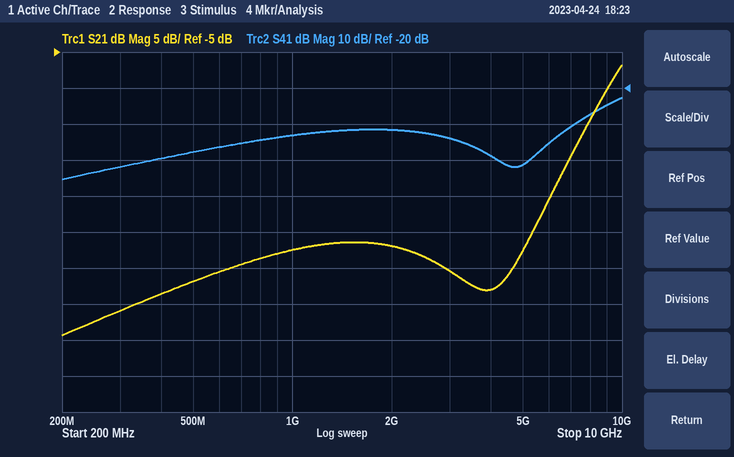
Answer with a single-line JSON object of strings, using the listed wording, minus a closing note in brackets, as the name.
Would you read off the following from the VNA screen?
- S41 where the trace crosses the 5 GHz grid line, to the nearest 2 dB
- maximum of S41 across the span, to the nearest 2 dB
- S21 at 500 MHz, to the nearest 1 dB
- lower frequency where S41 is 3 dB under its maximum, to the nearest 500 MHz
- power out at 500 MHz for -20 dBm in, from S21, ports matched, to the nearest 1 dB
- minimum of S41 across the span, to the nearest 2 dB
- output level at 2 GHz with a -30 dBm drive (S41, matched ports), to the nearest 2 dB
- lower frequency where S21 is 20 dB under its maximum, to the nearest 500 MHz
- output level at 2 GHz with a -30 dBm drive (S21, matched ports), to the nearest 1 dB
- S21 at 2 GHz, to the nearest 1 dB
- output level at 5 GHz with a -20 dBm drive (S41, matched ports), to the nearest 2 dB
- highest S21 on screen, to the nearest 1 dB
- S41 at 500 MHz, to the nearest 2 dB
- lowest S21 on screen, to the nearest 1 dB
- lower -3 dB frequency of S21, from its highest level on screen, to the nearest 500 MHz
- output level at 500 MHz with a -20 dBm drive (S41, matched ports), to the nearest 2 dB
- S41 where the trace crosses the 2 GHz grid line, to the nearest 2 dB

{"S41 where the trace crosses the 5 GHz grid line, to the nearest 2 dB": "-42 dB", "maximum of S41 across the span, to the nearest 2 dB": "-22 dB", "S21 at 500 MHz, to the nearest 1 dB": "-37 dB", "lower frequency where S41 is 3 dB under its maximum, to the nearest 500 MHz": "8.5 GHz", "power out at 500 MHz for -20 dBm in, from S21, ports matched, to the nearest 1 dB": "-57 dBm", "minimum of S41 across the span, to the nearest 2 dB": "-46 dB", "output level at 2 GHz with a -30 dBm drive (S41, matched ports), to the nearest 2 dB": "-62 dBm", "lower frequency where S21 is 20 dB under its maximum, to the nearest 500 MHz": "6.0 GHz", "output level at 2 GHz with a -30 dBm drive (S21, matched ports), to the nearest 1 dB": "-62 dBm", "S21 at 2 GHz, to the nearest 1 dB": "-32 dB", "output level at 5 GHz with a -20 dBm drive (S41, matched ports), to the nearest 2 dB": "-62 dBm", "highest S21 on screen, to the nearest 1 dB": "-7 dB", "S41 at 500 MHz, to the nearest 2 dB": "-38 dB", "lowest S21 on screen, to the nearest 1 dB": "-44 dB", "lower -3 dB frequency of S21, from its highest level on screen, to the nearest 500 MHz": "9.0 GHz", "output level at 500 MHz with a -20 dBm drive (S41, matched ports), to the nearest 2 dB": "-58 dBm", "S41 where the trace crosses the 2 GHz grid line, to the nearest 2 dB": "-32 dB"}
